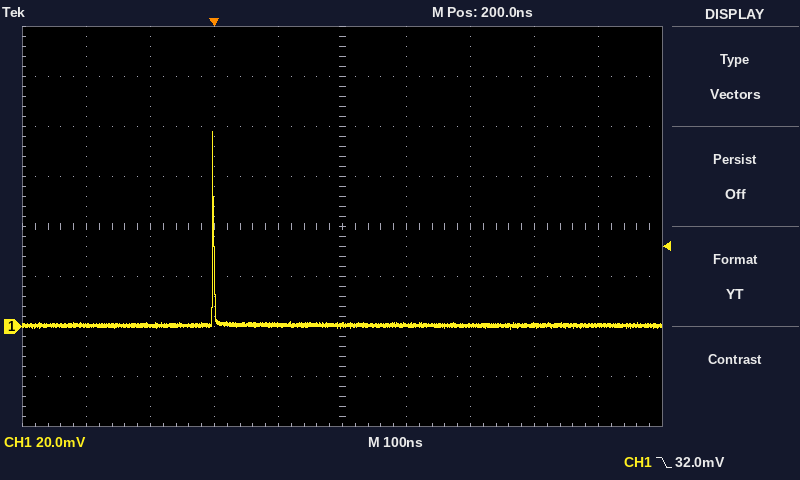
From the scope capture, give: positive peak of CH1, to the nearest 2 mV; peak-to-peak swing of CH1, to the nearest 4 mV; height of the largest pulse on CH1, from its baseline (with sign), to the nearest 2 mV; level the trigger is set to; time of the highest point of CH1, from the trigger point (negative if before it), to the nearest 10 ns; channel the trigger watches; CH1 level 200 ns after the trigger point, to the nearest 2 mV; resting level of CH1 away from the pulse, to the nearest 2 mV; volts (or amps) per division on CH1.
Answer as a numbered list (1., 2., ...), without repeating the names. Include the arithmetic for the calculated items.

1. 78 mV
2. 80 mV
3. 78 mV − (0 mV) = +78 mV
4. 32.0 mV
5. 0 ns
6. CH1
7. 0 mV
8. 0 mV
9. 20 mV
